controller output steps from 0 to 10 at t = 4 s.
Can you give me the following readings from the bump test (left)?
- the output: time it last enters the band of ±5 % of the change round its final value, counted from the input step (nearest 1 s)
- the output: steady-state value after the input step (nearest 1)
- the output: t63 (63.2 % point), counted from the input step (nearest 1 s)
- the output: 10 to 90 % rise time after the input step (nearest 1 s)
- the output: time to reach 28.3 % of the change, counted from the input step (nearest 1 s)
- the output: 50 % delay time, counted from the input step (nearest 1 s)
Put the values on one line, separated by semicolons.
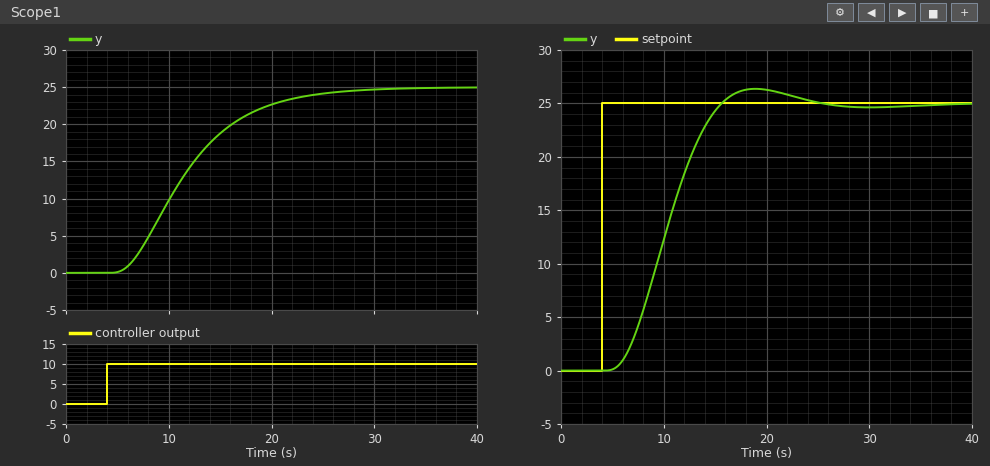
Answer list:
19 s; 25; 9 s; 13 s; 5 s; 7 s
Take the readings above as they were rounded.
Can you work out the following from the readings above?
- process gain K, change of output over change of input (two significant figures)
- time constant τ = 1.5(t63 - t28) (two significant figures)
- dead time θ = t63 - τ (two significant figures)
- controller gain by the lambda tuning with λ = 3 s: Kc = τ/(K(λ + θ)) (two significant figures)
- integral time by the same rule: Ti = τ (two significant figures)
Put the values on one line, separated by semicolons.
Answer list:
2.5; 6.0 s; 3.0 s; 0.40; 6.0 s
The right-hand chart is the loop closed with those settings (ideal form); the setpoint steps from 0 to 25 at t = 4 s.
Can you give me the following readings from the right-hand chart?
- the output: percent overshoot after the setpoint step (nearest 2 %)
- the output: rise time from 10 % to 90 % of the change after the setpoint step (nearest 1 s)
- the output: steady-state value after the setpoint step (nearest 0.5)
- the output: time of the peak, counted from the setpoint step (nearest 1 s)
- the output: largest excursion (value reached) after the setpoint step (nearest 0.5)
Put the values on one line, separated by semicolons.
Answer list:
6 %; 7 s; 25.0; 15 s; 26.5
